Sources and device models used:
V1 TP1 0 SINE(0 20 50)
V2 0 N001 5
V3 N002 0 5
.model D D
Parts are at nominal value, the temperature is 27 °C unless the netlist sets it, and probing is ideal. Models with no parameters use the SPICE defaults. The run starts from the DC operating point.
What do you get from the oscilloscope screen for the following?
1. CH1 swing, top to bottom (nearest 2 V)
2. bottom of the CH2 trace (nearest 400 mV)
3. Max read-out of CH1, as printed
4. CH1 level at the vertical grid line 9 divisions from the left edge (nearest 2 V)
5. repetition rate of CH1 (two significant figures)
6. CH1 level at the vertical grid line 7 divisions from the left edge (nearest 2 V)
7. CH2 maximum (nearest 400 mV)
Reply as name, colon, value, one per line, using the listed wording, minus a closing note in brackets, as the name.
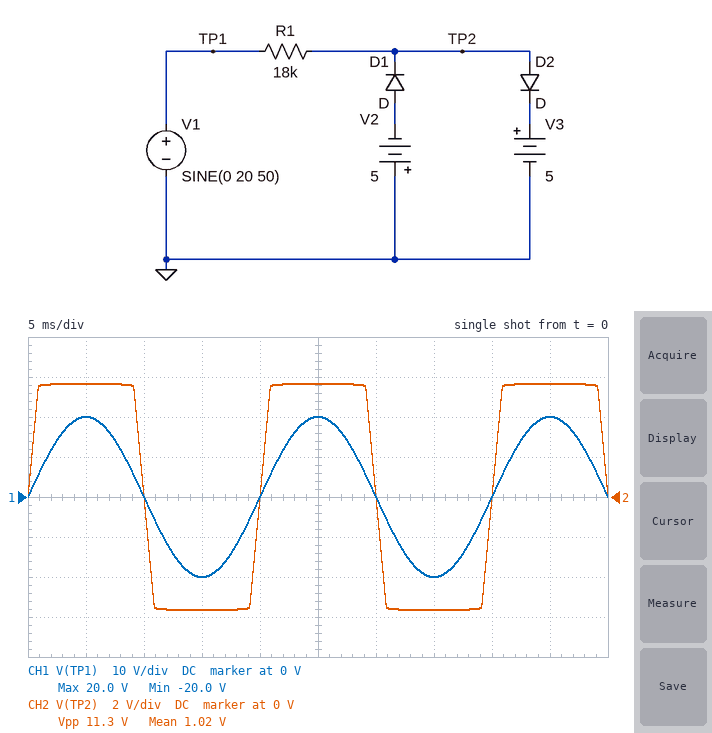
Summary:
CH1 swing, top to bottom: 40 V
bottom of the CH2 trace: -5.6 V
Max read-out of CH1, as printed: 20.0 V
CH1 level at the vertical grid line 9 divisions from the left edge: 20 V
repetition rate of CH1: 50 Hz
CH1 level at the vertical grid line 7 divisions from the left edge: -20 V
CH2 maximum: 5.6 V
